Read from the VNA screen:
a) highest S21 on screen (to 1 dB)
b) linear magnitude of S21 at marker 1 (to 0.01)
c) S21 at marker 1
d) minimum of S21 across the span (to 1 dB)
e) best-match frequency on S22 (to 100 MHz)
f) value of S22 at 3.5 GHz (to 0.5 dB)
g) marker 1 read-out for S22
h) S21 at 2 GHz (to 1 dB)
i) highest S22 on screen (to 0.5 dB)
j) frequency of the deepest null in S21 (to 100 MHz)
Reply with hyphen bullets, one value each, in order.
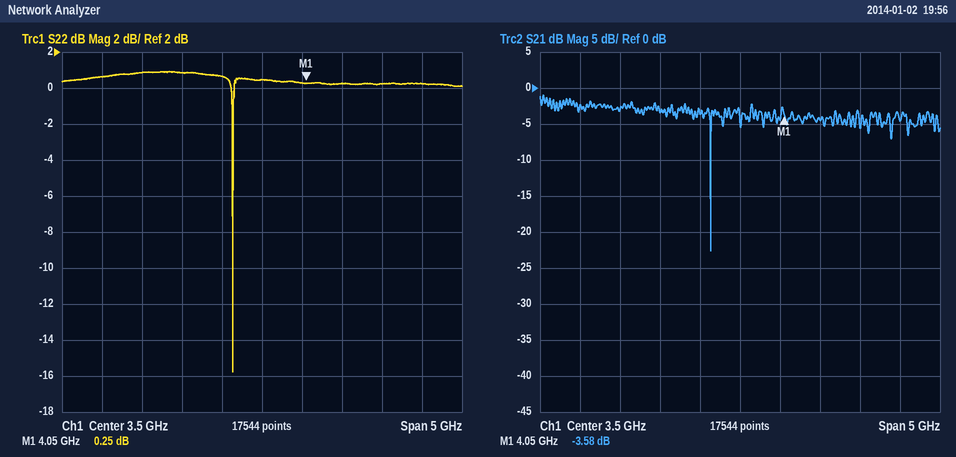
- -1 dB
- 0.66
- -3.58 dB
- -23 dB
- 3.1 GHz
- 0.5 dB
- 0.25 dB
- -3 dB
- 1.0 dB
- 3.1 GHz
